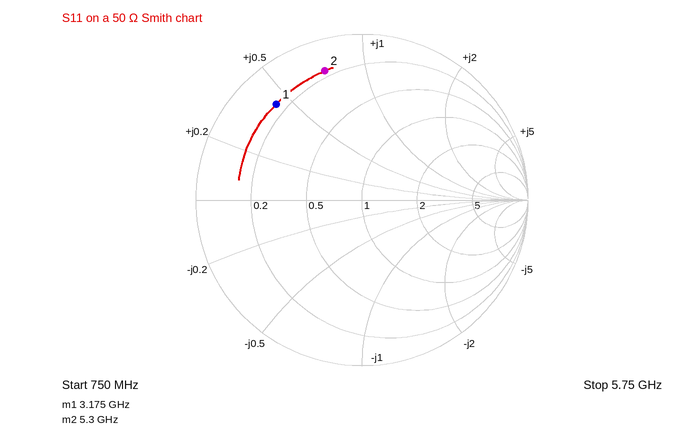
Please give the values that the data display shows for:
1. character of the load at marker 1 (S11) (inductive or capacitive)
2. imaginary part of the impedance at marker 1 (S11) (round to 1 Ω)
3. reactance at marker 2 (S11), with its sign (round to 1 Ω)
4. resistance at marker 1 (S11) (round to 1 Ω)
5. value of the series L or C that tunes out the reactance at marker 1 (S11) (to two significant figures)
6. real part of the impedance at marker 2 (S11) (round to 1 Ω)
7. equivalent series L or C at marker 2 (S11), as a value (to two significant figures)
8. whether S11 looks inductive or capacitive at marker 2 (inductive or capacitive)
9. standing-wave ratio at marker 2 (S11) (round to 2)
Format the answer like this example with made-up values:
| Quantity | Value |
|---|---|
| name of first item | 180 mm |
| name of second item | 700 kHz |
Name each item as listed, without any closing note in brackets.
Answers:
| Quantity | Value |
|---|---|
| character of the load at marker 1 (S11) | inductive |
| imaginary part of the impedance at marker 1 (S11) | +22 Ω |
| reactance at marker 2 (S11), with its sign | +37 Ω |
| resistance at marker 1 (S11) | 8 Ω |
| value of the series L or C that tunes out the reactance at marker 1 (S11) | 2.3 pF |
| real part of the impedance at marker 2 (S11) | 8 Ω |
| equivalent series L or C at marker 2 (S11), as a value | 1.1 nH |
| whether S11 looks inductive or capacitive at marker 2 | inductive |
| standing-wave ratio at marker 2 (S11) | 10 |
